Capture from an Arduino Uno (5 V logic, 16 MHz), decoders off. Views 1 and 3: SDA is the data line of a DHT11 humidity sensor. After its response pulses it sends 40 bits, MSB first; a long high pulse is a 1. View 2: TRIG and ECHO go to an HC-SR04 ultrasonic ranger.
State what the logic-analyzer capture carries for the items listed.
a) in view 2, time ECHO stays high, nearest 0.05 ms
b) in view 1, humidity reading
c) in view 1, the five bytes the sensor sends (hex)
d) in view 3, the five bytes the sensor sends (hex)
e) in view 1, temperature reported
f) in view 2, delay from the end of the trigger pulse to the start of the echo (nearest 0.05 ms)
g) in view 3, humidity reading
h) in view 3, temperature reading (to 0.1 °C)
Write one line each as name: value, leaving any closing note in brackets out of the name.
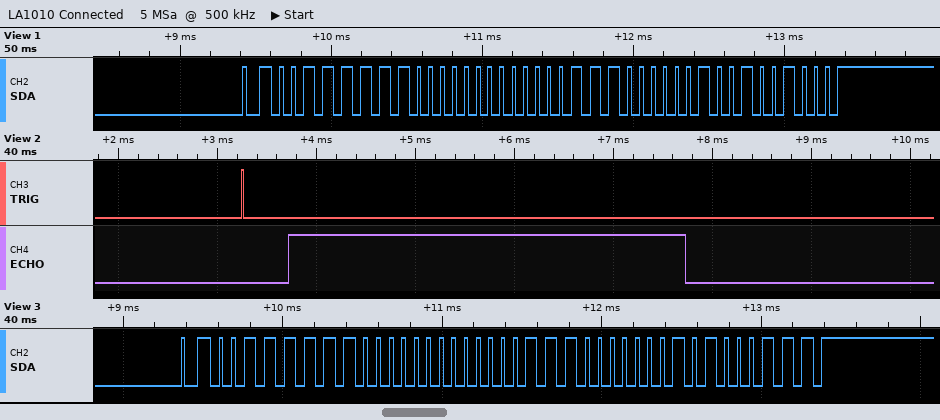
in view 2, time ECHO stays high, nearest 0.05 ms: 4.00 ms
in view 1, humidity reading: 63 %
in view 1, the five bytes the sensor sends: 3F 00 07 02 48
in view 3, the five bytes the sensor sends: 3F 00 07 01 47
in view 1, temperature reported: 7.2 °C
in view 2, delay from the end of the trigger pulse to the start of the echo: 0.45 ms
in view 3, humidity reading: 63 %
in view 3, temperature reading: 7.1 °C
